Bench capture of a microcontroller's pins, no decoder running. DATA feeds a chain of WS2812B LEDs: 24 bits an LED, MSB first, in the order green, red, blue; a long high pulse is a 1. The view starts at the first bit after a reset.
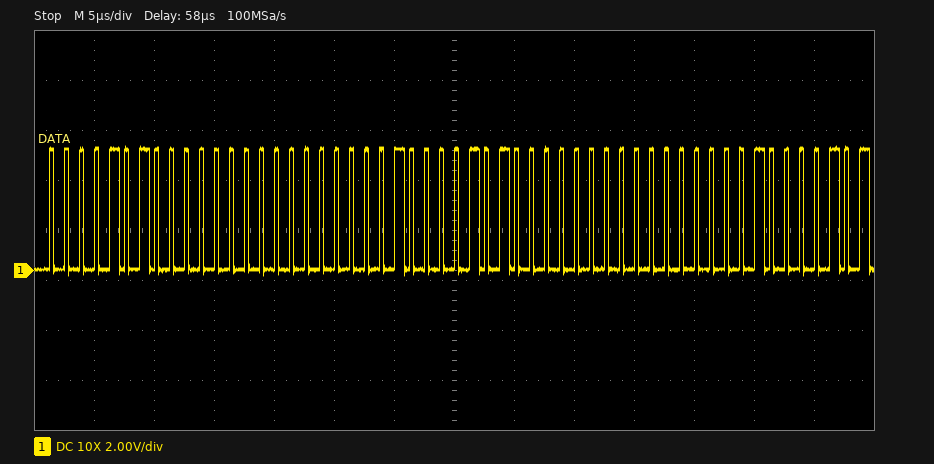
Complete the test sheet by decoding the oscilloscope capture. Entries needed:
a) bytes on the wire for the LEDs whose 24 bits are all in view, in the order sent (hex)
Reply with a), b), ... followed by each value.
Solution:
a) 0A 00 01 0A 00 01
